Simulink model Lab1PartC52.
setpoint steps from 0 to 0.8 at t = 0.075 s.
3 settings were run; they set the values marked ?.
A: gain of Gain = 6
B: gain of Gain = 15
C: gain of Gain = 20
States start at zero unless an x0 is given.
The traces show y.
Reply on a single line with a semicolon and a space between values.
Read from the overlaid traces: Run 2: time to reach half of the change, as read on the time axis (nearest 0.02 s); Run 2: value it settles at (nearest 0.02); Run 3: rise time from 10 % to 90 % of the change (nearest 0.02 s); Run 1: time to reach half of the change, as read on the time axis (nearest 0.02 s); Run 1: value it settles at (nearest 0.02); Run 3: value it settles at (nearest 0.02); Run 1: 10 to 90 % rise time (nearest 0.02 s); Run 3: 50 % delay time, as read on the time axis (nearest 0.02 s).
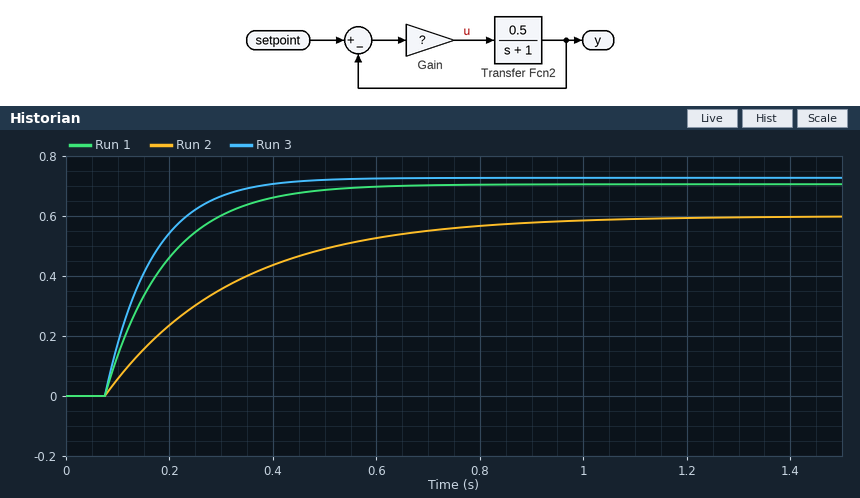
0.24 s; 0.60; 0.20 s; 0.16 s; 0.70; 0.72; 0.26 s; 0.14 s
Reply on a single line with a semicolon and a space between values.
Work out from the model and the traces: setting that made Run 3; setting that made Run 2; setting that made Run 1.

C; A; B
